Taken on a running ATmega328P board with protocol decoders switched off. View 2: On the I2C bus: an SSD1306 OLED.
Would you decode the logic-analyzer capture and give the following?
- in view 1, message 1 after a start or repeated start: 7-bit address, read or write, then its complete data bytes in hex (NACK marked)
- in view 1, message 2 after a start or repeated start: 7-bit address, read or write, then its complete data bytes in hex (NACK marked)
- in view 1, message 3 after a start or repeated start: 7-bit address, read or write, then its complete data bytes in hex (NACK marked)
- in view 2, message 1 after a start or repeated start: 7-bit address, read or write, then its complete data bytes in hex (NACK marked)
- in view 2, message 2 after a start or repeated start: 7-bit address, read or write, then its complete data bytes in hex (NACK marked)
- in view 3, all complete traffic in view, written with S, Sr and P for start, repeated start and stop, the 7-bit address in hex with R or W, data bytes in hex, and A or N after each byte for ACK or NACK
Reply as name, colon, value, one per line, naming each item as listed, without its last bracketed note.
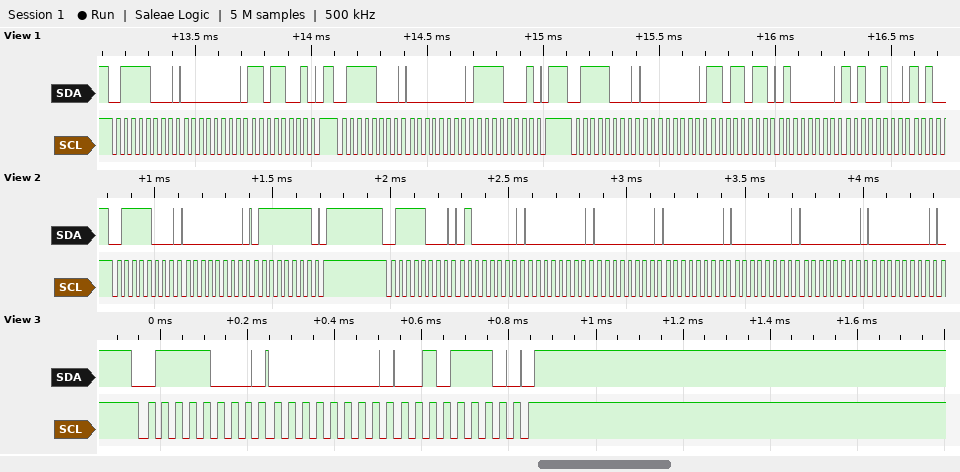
in view 1, message 1 after a start or repeated start: 7-bit address, read or write, then its complete data bytes in hex: 0x3C write: 00 D9
in view 1, message 2 after a start or repeated start: 7-bit address, read or write, then its complete data bytes in hex: 0x3C write: 00 F1
in view 1, message 3 after a start or repeated start: 7-bit address, read or write, then its complete data bytes in hex: 0x3C write: 00 DB 40 A4
in view 2, message 1 after a start or repeated start: 7-bit address, read or write, then its complete data bytes in hex: 0x3C write: 00 7F
in view 2, message 2 after a start or repeated start: 7-bit address, read or write, then its complete data bytes in hex: 0x3C write: 40 00 00 00 00 00 00
in view 3, all complete traffic in view, written with S, Sr and P for start, repeated start and stop, the 7-bit address in hex with R or W, data bytes in hex, and A or N after each byte for ACK or NACK: S 3CW A 00 A 2E A P
